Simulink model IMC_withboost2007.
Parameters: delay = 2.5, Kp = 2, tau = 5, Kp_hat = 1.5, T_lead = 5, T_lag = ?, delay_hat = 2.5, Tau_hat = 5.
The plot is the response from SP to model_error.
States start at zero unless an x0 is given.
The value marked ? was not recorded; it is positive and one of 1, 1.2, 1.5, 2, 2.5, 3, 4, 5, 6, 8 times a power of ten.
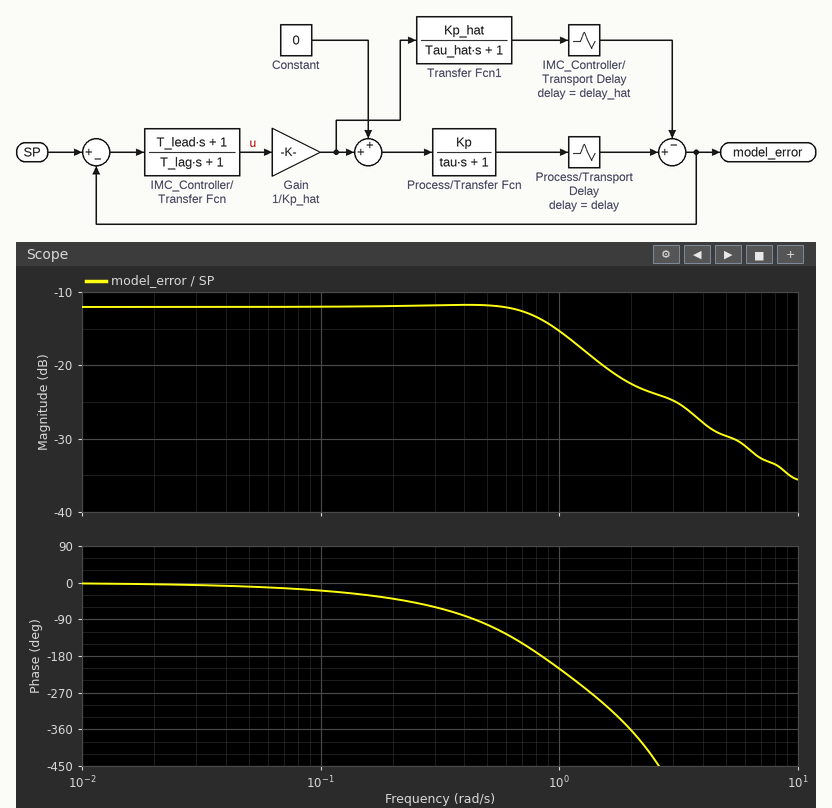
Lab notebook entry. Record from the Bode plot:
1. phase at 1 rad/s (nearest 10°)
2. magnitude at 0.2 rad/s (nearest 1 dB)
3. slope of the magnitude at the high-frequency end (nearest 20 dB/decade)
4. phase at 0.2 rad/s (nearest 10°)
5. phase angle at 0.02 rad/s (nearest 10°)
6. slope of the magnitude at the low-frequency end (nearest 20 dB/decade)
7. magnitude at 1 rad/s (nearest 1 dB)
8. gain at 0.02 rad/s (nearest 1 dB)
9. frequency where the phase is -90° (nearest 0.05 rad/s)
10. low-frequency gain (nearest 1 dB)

-210°
-12 dB
-20 dB/decade
-40°
0°
0 dB/decade
-15 dB
-12 dB
0.45 rad/s
-12 dB
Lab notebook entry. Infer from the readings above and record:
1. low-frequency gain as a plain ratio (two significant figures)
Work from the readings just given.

0.25
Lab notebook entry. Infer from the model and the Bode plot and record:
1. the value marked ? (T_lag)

2
